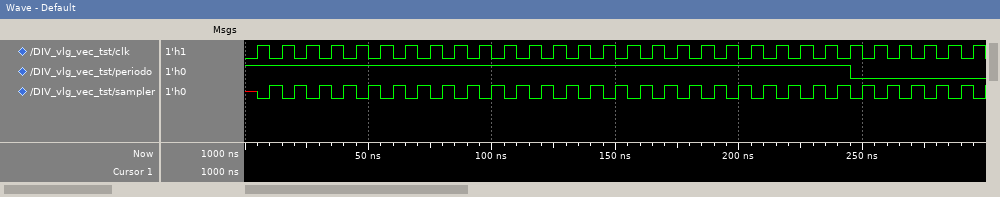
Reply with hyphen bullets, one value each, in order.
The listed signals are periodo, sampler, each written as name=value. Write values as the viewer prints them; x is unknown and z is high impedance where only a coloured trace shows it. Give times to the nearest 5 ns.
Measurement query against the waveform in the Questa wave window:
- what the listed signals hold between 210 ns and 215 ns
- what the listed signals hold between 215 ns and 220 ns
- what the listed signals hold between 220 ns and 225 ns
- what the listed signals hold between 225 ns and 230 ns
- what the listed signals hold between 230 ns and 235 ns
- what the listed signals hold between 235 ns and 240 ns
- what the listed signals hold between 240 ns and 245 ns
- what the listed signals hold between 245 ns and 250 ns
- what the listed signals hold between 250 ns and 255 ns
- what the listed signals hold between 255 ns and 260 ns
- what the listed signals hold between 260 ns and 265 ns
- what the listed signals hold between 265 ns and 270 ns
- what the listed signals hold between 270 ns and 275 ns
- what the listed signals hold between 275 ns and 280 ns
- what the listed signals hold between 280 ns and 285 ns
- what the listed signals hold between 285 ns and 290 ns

- periodo=1, sampler=1
- periodo=1, sampler=0
- periodo=1, sampler=1
- periodo=1, sampler=0
- periodo=1, sampler=1
- periodo=1, sampler=0
- periodo=1, sampler=1
- periodo=0, sampler=0
- periodo=0, sampler=1
- periodo=0, sampler=0
- periodo=0, sampler=1
- periodo=0, sampler=0
- periodo=0, sampler=1
- periodo=0, sampler=0
- periodo=0, sampler=1
- periodo=0, sampler=0
